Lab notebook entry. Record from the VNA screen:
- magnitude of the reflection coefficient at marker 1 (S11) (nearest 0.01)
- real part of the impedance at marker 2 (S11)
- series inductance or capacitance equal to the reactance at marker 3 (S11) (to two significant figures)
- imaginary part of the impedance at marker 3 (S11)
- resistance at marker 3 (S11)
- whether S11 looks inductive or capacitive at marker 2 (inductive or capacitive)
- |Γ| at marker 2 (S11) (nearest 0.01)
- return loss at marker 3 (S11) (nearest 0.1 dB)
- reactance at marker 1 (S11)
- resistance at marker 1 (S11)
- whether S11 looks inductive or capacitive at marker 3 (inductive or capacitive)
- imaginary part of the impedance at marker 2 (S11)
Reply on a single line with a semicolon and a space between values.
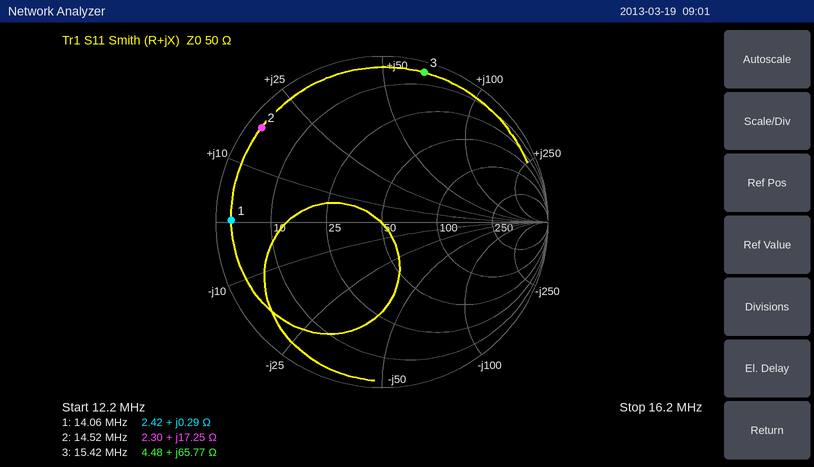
0.91; 2.30 Ω; 680 nH; +65.77 Ω; 4.48 Ω; inductive; 0.92; 0.6 dB; +0.29 Ω; 2.42 Ω; inductive; +17.25 Ω
